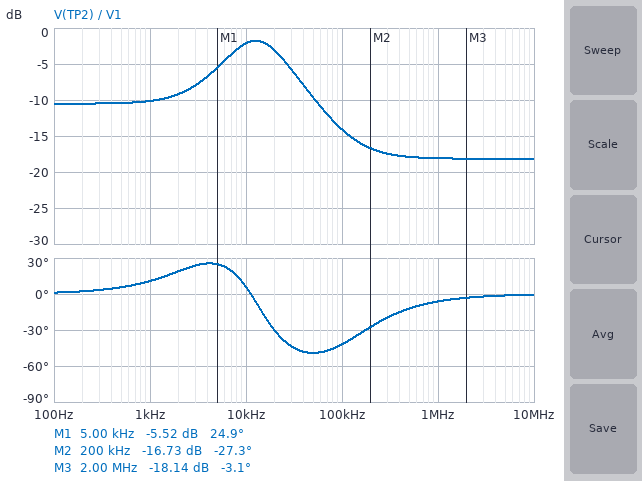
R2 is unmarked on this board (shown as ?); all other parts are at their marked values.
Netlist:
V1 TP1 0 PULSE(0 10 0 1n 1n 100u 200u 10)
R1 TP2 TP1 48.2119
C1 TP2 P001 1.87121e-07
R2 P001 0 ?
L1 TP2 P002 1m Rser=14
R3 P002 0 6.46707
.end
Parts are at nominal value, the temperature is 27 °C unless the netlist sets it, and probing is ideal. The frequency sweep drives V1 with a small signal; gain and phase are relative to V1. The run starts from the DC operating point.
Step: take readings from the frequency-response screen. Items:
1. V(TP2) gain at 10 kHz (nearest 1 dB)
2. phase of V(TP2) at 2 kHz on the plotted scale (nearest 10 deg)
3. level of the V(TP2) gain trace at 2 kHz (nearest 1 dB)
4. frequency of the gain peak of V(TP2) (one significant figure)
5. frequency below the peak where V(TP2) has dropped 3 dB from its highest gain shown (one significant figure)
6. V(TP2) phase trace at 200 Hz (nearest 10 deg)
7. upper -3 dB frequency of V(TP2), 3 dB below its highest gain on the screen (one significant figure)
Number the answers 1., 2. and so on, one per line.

1. -2 dB
2. 20 deg
3. -9 dB
4. 10 kHz
5. 6 kHz
6. 0 deg
7. 30 kHz
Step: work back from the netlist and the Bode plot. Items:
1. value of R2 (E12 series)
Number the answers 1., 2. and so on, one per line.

1. 6.8 Ω
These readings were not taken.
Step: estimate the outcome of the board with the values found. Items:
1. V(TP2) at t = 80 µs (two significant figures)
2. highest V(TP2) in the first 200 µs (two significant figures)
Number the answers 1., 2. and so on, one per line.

1. 2.9 V
2. 6.4 V
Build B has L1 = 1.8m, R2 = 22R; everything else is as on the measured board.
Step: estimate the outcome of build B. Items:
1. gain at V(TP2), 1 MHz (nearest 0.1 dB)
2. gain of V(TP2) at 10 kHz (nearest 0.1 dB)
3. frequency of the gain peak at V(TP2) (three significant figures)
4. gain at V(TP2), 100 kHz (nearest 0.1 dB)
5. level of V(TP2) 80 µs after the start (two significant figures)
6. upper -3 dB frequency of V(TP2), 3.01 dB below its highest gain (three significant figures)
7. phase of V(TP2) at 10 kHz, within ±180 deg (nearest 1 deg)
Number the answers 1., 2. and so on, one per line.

1. -10.1 dB
2. -1.7 dB
3. 8.61 kHz
4. -9.5 dB
5. 3.4 V
6. 21.5 kHz
7. -6 deg
